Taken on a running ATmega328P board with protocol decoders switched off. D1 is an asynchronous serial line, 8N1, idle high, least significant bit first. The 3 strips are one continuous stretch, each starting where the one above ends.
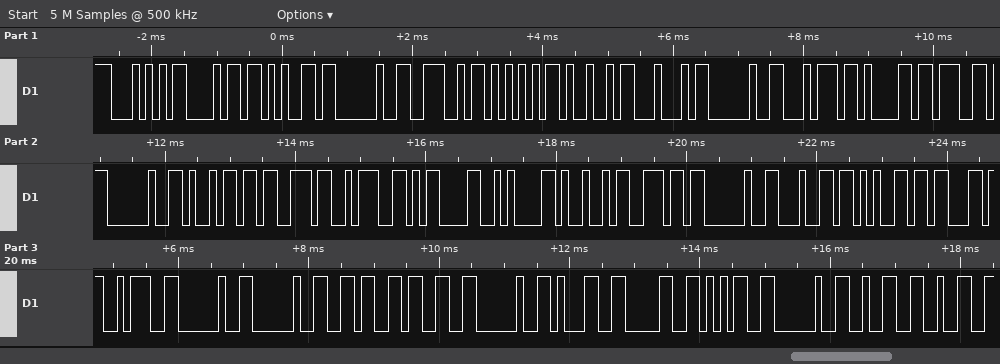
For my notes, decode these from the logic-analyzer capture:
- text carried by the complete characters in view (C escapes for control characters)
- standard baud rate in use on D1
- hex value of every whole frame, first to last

"The NUID tag is:\r\nIn dec:  63 105 22"
9600 baud
54 68 65 20 4E 55 49 44 20 74 61 67 20 69 73 3A 0D 0A 49 6E 20 64 65 63 3A 20 20 36 33 20 31 30 35 20 32 32
